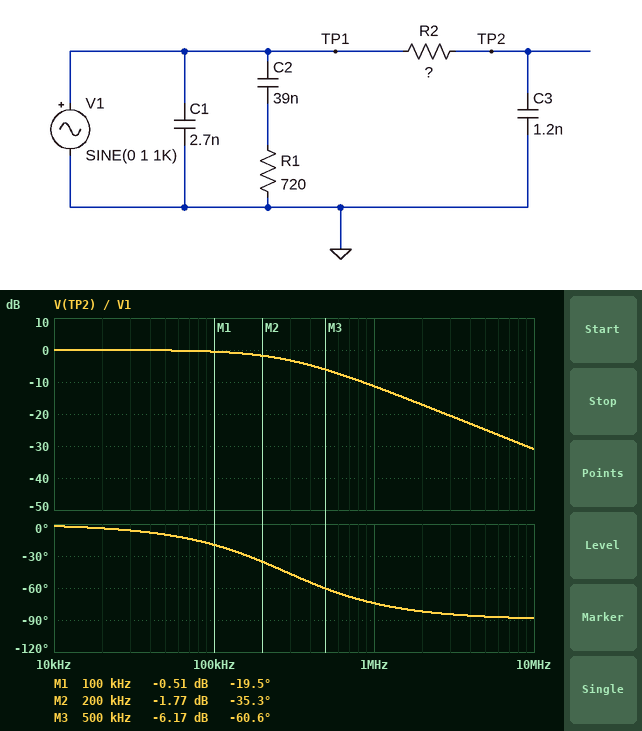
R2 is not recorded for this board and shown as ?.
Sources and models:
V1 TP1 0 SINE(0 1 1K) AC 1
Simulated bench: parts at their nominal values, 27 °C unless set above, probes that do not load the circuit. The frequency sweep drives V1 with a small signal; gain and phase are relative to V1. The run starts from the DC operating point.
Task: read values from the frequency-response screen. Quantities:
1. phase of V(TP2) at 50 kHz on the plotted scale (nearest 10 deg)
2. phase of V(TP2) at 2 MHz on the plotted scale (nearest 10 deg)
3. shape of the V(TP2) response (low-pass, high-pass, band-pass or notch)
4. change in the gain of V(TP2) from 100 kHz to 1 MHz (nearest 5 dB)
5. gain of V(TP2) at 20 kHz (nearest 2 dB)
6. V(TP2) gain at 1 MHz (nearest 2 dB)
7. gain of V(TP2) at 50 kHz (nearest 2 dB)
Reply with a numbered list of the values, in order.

1. -10 deg
2. -80 deg
3. low-pass
4. -10 dB
5. 0 dB
6. -12 dB
7. 0 dB
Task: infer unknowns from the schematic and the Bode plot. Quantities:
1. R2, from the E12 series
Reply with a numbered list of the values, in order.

1. 470 Ω
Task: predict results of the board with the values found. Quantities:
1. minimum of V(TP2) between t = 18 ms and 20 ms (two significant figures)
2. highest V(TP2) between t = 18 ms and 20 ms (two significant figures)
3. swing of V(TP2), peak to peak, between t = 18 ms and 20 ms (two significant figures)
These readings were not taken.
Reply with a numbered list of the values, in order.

1. -1.0 V
2. 1.0 V
3. 2.0 V
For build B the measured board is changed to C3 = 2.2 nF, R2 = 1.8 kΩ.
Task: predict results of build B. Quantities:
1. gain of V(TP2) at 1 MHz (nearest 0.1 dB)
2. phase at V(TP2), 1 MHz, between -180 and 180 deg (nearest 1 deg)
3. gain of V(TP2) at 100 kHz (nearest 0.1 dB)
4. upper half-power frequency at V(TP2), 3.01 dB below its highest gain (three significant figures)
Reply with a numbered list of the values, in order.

1. -27.9 dB
2. -88 deg
3. -8.6 dB
4. 40.2 kHz
